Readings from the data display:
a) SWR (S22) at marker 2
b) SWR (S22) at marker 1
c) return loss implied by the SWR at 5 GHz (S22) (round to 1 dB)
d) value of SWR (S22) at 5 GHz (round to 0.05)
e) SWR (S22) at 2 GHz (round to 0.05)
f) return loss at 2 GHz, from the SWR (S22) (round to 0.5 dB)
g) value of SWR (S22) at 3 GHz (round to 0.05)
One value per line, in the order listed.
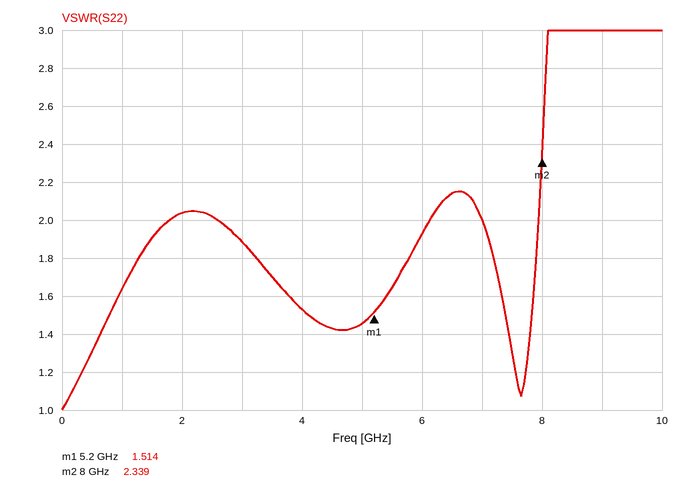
2.339
1.514
15 dB
1.45
2.05
9.5 dB
1.90
